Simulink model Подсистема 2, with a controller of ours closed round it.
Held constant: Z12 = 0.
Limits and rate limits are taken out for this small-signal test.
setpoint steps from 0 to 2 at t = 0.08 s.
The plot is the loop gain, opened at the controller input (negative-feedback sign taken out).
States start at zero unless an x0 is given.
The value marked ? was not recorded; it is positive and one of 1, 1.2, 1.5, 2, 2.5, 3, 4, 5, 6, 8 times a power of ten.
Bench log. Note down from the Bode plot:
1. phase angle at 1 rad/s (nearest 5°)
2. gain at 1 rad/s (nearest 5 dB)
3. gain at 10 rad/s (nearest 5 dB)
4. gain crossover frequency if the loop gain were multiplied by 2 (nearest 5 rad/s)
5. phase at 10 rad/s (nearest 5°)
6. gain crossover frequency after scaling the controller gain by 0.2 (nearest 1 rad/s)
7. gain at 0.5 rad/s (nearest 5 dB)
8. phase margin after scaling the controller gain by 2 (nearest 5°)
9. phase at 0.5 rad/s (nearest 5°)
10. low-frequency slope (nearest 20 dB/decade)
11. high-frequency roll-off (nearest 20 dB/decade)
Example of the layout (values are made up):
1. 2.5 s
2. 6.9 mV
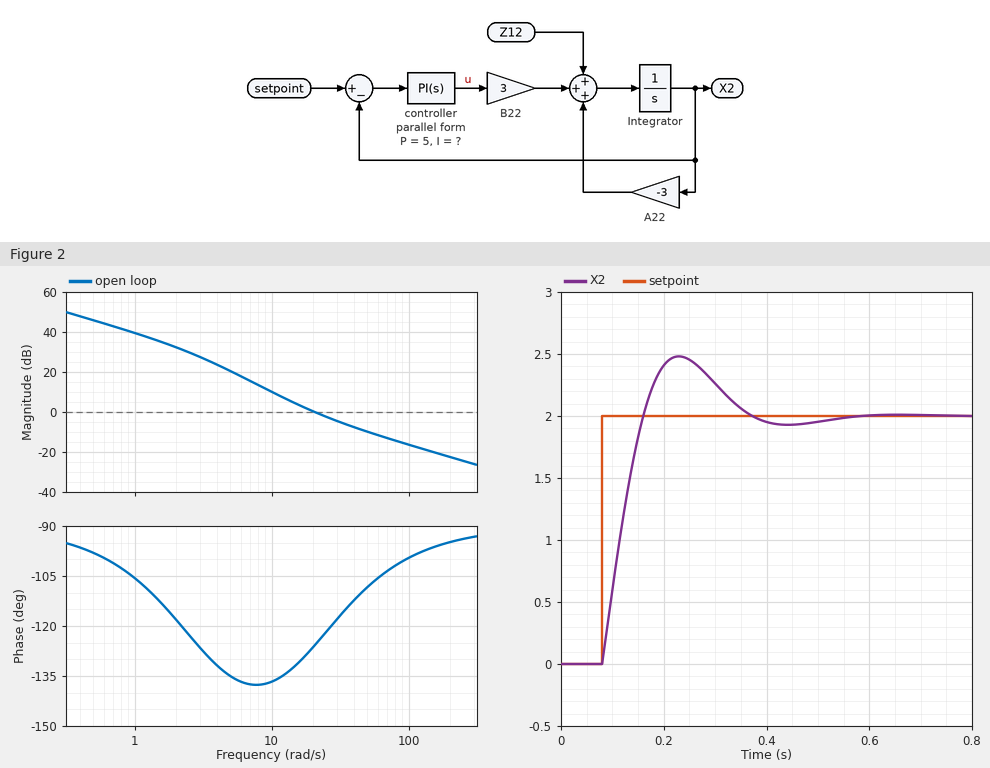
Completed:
1. -105°
2. 40 dB
3. 10 dB
4. 35 rad/s
5. -135°
6. 8 rad/s
7. 45 dB
8. 65°
9. -100°
10. -20 dB/decade
11. -20 dB/decade
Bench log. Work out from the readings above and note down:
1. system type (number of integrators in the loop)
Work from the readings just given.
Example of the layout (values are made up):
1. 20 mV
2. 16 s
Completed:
1. 1
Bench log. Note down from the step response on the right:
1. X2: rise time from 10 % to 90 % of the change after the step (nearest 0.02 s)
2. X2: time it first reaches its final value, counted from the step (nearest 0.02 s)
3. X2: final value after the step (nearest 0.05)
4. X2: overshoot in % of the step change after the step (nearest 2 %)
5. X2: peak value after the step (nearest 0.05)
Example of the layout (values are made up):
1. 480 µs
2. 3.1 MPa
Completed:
1. 0.06 s
2. 0.08 s
3. 2.00
4. 24 %
5. 2.50
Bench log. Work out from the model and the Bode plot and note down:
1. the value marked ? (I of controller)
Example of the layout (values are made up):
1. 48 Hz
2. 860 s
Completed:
1. 100
